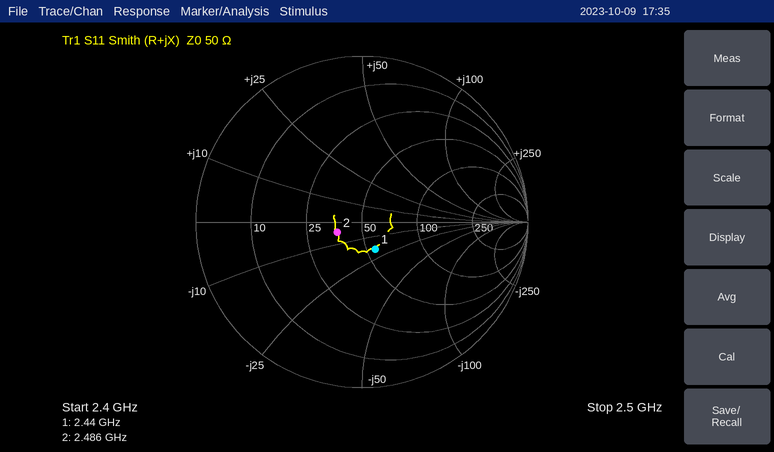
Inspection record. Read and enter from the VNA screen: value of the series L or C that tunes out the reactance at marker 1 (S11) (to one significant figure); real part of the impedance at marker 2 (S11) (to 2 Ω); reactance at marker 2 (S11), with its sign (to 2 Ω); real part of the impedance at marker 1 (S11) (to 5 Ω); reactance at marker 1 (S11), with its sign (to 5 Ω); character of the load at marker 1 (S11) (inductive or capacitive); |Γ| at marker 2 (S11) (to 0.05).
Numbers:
1 nH
36 Ω
-4 Ω
55 Ω
-20 Ω
capacitive
0.15
